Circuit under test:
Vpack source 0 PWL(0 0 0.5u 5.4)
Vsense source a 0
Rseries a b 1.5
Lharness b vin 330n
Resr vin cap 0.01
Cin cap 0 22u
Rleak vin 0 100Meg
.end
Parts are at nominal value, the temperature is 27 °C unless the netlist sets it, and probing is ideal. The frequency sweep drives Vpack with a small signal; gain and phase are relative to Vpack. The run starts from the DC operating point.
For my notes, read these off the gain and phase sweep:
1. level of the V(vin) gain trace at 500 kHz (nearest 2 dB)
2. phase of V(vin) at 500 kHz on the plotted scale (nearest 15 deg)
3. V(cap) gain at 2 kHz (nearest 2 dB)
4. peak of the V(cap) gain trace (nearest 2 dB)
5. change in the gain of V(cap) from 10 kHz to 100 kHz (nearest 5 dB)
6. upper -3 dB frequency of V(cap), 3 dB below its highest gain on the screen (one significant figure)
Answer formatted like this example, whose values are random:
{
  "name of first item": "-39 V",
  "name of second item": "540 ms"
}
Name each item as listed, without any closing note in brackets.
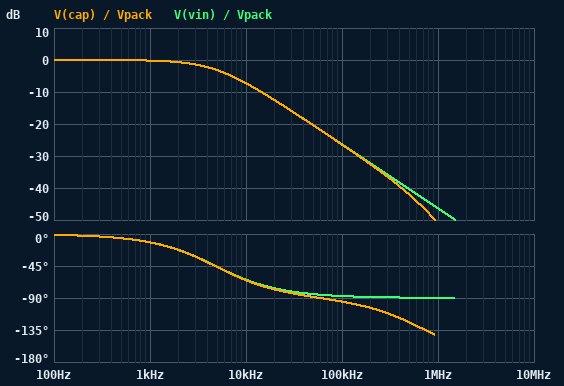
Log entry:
{
  "level of the V(vin) gain trace at 500 kHz": "-40 dB",
  "phase of V(vin) at 500 kHz on the plotted scale": "-90 deg",
  "V(cap) gain at 2 kHz": "0 dB",
  "peak of the V(cap) gain trace": "0 dB",
  "change in the gain of V(cap) from 10 kHz to 100 kHz": "-20 dB",
  "upper -3 dB frequency of V(cap), 3 dB below its highest gain on the screen": "5 kHz"
}
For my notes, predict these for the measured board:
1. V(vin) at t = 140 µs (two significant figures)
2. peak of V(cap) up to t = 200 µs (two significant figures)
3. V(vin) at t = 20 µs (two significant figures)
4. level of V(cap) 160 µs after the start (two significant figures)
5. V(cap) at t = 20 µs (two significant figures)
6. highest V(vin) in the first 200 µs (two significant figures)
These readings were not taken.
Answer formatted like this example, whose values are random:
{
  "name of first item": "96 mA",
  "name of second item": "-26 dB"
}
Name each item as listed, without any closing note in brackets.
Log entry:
{
  "V(vin) at t = 140 µs": "5.3 V",
  "peak of V(cap) up to t = 200 µs": "5.4 V",
  "V(vin) at t = 20 µs": "2.4 V",
  "level of V(cap) 160 µs after the start": "5.4 V",
  "V(cap) at t = 20 µs": "2.4 V",
  "highest V(vin) in the first 200 µs": "5.4 V"
}
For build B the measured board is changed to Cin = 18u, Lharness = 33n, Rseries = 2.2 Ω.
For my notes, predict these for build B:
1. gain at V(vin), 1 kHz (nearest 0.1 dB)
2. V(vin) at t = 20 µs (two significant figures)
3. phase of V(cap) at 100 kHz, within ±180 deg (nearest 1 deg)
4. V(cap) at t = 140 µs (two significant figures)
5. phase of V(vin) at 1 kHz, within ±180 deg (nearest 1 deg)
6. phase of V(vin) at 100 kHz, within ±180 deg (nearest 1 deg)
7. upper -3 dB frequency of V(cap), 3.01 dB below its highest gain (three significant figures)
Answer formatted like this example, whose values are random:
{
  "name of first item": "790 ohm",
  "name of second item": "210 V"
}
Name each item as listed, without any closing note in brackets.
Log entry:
{
  "gain at V(vin), 1 kHz": "-0.3 dB",
  "V(vin) at t = 20 µs": "2.1 V",
  "phase of V(cap) at 100 kHz, within ±180 deg": "-88 deg",
  "V(cap) at t = 140 µs": "5.2 V",
  "phase of V(vin) at 1 kHz, within ±180 deg": "-14 deg",
  "phase of V(vin) at 100 kHz, within ±180 deg": "-82 deg",
  "upper -3 dB frequency of V(cap), 3.01 dB below its highest gain": "4.00 kHz"
}
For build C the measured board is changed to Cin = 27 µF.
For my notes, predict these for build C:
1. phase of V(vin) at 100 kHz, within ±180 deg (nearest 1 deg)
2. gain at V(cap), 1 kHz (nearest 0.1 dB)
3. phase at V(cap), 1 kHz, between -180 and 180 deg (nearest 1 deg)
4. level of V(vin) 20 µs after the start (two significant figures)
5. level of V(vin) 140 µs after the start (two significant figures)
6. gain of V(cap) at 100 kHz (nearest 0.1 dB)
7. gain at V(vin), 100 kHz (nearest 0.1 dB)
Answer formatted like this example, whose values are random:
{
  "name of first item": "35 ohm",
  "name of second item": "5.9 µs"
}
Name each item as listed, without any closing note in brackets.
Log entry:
{
  "phase of V(vin) at 100 kHz, within ±180 deg": "-86 deg",
  "gain at V(cap), 1 kHz": "-0.3 dB",
  "phase at V(cap), 1 kHz, between -180 and 180 deg": "-14 deg",
  "level of V(vin) 20 µs after the start": "2.1 V",
  "level of V(vin) 140 µs after the start": "5.2 V",
  "gain of V(cap) at 100 kHz": "-28.2 dB",
  "gain at V(vin), 100 kHz": "-28.1 dB"
}
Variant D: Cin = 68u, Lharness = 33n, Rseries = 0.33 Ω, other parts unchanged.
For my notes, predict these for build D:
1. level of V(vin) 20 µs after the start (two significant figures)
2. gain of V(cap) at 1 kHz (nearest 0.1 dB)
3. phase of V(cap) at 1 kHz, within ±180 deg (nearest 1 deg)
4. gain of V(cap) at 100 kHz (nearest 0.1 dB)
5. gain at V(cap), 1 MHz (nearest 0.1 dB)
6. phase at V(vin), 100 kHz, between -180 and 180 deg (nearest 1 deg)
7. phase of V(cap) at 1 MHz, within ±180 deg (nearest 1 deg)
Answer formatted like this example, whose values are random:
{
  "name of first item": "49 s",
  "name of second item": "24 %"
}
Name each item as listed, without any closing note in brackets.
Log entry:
{
  "level of V(vin) 20 µs after the start": "3.2 V",
  "gain of V(cap) at 1 kHz": "-0.1 dB",
  "phase of V(cap) at 1 kHz, within ±180 deg": "-8 deg",
  "gain of V(cap) at 100 kHz": "-23.2 dB",
  "gain at V(cap), 1 MHz": "-44.6 dB",
  "phase at V(vin), 100 kHz, between -180 and 180 deg": "-66 deg",
  "phase of V(cap) at 1 MHz, within ±180 deg": "-121 deg"
}
